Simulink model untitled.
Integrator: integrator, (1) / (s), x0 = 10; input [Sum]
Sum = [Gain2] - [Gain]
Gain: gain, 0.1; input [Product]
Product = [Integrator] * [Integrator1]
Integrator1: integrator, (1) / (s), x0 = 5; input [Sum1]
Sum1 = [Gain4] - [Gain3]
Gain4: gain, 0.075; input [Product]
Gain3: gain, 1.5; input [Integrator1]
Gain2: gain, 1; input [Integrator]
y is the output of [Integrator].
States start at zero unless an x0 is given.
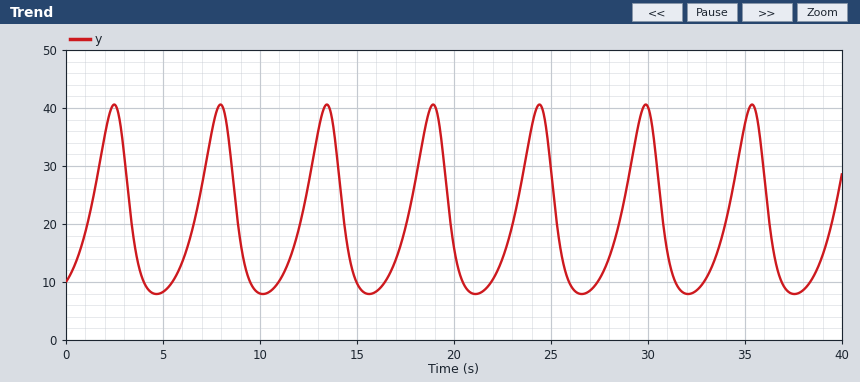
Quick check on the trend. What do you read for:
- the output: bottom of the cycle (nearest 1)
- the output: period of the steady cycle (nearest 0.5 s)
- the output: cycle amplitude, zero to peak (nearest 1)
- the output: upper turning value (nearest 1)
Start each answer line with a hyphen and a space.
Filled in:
- 8
- 5.5 s
- 16
- 41
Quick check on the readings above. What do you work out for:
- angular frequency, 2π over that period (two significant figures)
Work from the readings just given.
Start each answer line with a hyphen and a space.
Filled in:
- 1.1 rad/s
